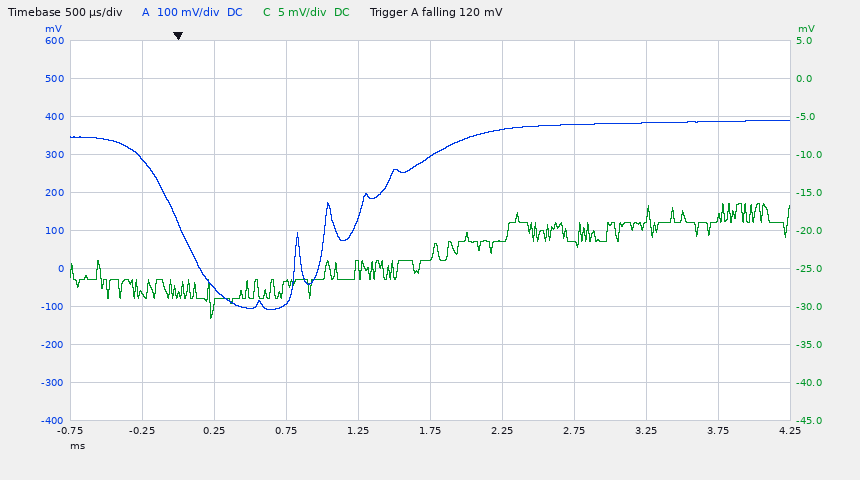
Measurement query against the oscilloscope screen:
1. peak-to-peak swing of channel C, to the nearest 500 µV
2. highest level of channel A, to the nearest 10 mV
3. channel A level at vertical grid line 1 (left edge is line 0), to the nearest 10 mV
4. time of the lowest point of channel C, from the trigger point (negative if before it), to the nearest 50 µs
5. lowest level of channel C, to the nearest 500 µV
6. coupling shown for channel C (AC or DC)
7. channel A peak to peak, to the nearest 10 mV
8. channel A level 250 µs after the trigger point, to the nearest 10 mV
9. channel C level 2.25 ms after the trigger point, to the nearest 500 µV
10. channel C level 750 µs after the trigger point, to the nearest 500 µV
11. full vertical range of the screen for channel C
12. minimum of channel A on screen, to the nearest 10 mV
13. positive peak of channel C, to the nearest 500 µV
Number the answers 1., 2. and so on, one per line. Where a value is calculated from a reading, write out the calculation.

1. -16.5 mV − (-31.5 mV) = 15.0 mV
2. 390 mV
3. 290 mV
4. +250 µs
5. -31.5 mV
6. DC
7. 390 mV − (-110 mV) = 500 mV
8. -50 mV
9. -21.5 mV
10. -27.0 mV
11. 50 mV
12. -110 mV
13. -16.5 mV
